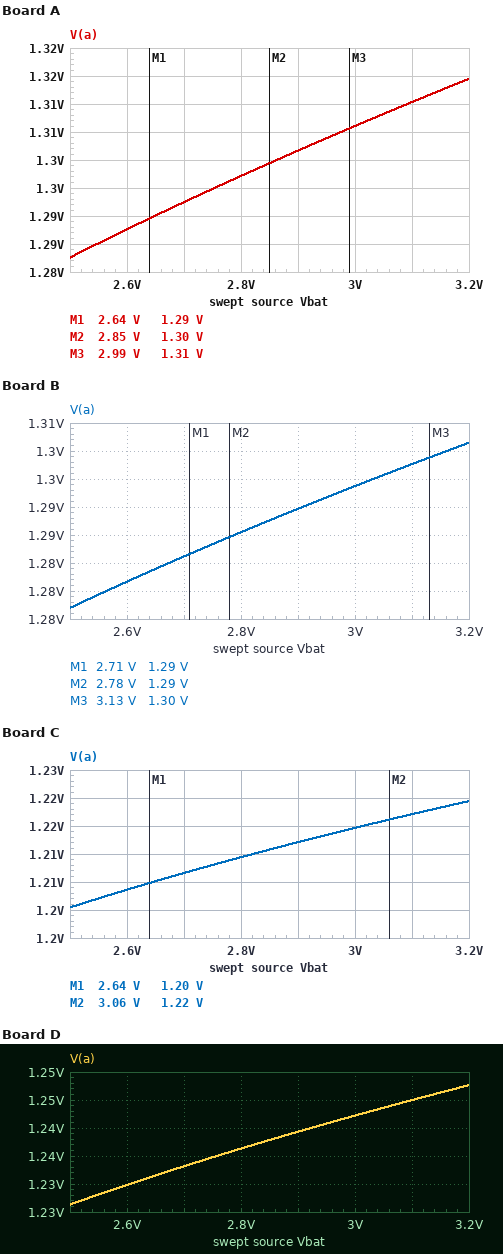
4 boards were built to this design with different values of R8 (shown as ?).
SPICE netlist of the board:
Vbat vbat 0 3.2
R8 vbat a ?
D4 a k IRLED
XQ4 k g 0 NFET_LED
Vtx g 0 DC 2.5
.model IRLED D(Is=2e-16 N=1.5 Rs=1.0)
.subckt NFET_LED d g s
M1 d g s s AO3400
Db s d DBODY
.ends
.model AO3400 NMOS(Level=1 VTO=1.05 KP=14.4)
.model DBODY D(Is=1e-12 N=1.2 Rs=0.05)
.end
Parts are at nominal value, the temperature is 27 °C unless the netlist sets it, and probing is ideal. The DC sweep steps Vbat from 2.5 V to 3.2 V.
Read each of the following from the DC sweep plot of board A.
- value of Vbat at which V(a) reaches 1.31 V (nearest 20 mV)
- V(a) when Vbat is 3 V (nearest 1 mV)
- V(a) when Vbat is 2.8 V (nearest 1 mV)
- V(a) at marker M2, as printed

2.98 V
1.311 V
1.302 V
1.30 V
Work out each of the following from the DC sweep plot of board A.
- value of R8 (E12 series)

47 Ω
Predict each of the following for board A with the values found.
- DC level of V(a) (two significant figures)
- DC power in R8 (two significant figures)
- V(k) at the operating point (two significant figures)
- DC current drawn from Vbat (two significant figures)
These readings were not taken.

1.3 V
75 mW
1.9 mV
40 mA
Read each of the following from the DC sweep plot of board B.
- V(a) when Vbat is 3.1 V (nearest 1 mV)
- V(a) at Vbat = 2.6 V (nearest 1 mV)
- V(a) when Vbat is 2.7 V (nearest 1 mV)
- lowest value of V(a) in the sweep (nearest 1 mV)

1.303 V
1.282 V
1.286 V
1.277 V
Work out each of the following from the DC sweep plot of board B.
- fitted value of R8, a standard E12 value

56 Ω
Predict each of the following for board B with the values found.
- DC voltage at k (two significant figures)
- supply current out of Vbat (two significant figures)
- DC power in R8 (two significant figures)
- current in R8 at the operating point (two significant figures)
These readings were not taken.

1.6 mV
34 mA
64 mW
34 mA
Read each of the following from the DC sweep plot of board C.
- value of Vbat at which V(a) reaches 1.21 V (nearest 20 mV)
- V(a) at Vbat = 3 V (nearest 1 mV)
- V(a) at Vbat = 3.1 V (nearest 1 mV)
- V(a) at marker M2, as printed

2.64 V
1.215 V
1.217 V
1.22 V
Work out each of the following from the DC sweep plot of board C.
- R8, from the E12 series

270 Ω
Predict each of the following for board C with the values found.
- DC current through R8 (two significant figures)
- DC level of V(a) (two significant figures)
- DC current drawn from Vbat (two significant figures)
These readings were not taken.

7.3 mA
1.2 V
7.3 mA
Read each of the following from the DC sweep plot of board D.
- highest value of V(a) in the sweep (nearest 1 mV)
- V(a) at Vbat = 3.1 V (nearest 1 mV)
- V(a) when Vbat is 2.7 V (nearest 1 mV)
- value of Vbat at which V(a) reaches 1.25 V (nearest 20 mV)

1.248 V
1.245 V
1.233 V
3.10 V
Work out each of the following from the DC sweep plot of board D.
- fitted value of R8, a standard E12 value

150 Ω
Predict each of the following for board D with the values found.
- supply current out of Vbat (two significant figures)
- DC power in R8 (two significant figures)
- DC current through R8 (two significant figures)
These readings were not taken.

13 mA
25 mW
13 mA
